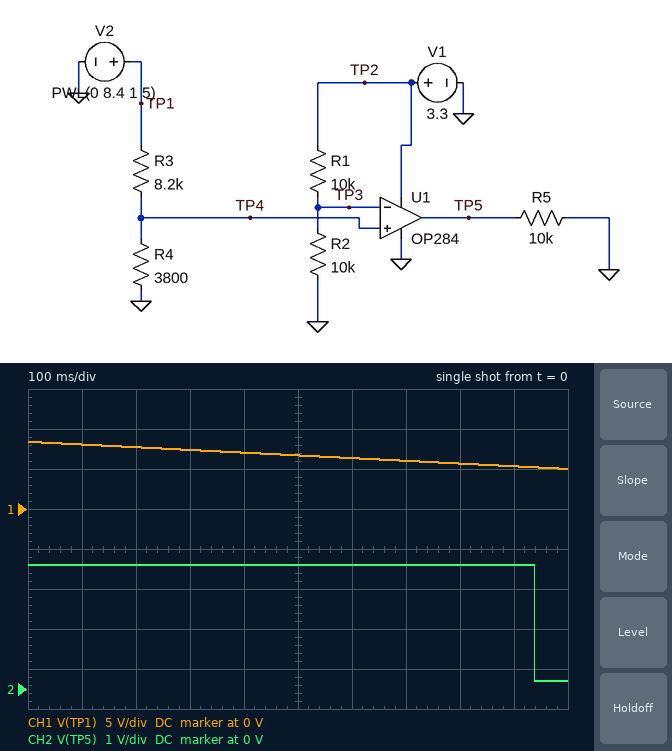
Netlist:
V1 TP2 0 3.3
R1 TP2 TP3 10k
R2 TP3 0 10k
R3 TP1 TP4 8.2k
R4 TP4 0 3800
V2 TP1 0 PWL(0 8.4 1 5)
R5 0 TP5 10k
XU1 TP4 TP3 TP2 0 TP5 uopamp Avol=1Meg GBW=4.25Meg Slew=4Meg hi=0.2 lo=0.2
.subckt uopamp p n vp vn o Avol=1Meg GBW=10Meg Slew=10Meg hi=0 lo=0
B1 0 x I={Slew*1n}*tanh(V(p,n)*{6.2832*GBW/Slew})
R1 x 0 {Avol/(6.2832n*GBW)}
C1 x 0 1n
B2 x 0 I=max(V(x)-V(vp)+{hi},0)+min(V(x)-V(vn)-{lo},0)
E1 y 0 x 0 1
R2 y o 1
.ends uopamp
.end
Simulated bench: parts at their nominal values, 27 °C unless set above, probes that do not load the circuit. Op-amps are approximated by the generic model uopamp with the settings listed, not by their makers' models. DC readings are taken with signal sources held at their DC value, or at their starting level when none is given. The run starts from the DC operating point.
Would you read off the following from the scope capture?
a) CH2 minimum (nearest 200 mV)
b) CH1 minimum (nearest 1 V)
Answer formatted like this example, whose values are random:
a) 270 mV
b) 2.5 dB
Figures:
a) 200 mV
b) 5 V
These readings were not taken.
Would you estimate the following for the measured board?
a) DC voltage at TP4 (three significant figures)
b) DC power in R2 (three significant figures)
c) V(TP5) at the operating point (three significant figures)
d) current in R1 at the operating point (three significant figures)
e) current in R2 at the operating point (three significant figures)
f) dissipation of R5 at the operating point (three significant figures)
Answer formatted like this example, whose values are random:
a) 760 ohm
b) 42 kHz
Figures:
a) 2.66 V
b) 272 µW
c) 3.10 V
d) 165 µA
e) 165 µA
f) 963 µW
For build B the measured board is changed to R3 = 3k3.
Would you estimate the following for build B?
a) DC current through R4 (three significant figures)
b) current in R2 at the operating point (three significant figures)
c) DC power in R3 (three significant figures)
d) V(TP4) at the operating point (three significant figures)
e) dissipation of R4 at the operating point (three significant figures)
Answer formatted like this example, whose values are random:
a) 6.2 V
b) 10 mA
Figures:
a) 1.18 mA
b) 165 µA
c) 4.62 mW
d) 4.50 V
e) 5.32 mW
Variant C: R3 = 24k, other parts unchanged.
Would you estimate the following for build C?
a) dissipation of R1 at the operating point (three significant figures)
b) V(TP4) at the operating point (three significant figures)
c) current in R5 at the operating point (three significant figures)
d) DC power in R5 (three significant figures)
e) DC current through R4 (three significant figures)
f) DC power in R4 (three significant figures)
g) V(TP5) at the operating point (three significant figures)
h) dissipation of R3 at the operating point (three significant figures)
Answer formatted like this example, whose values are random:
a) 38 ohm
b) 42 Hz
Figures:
a) 272 µW
b) 1.15 V
c) 19.6 µA
d) 3.84 µW
e) 302 µA
f) 347 µW
g) 196 mV
h) 2.19 mW
